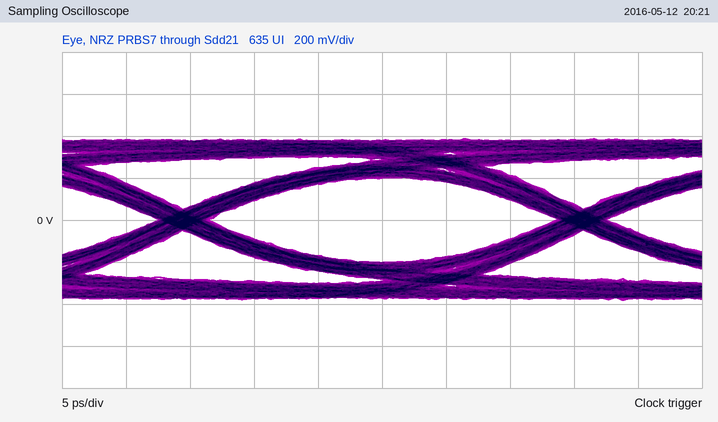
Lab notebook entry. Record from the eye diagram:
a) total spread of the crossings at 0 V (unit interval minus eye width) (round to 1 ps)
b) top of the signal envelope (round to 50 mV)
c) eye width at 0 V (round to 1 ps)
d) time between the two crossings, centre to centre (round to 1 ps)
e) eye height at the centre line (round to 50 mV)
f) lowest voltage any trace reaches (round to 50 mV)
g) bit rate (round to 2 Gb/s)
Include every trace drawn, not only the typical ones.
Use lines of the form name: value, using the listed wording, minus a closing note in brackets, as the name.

total spread of the crossings at 0 V (unit interval minus eye width): 4 ps
top of the signal envelope: 400 mV
eye width at 0 V: 27 ps
time between the two crossings, centre to centre: 31 ps
eye height at the centre line: 400 mV
lowest voltage any trace reaches: -400 mV
bit rate: 32 Gb/s
